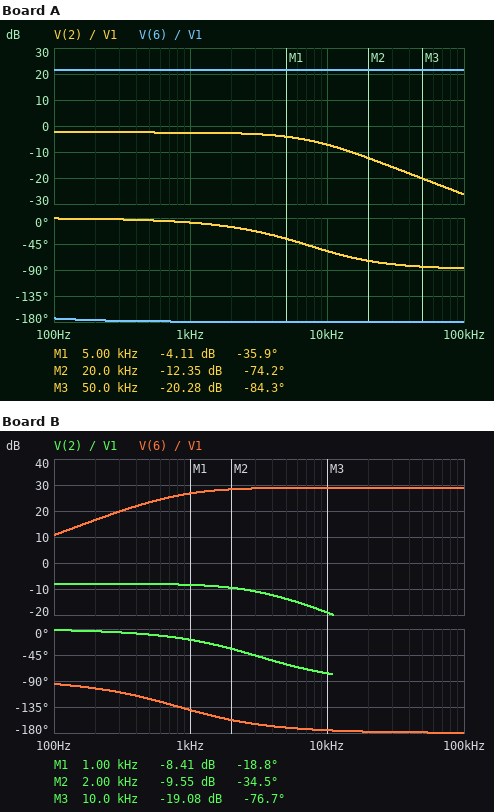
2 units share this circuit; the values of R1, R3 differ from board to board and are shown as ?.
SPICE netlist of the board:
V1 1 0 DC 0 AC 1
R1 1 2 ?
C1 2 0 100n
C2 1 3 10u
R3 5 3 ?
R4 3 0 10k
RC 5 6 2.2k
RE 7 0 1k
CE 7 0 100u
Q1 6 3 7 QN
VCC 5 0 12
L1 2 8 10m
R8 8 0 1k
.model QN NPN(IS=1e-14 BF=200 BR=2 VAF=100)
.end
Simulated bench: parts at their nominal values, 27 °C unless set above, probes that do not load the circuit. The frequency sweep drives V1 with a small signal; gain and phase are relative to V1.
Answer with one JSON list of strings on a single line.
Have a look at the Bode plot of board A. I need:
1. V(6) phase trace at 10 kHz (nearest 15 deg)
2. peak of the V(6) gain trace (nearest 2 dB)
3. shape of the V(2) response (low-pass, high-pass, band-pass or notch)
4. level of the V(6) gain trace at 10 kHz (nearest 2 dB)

["-180 deg", "22 dB", "low-pass", "22 dB"]
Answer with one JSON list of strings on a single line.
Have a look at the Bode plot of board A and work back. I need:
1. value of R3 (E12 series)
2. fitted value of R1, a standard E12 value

["150 kΩ", "330 Ω"]
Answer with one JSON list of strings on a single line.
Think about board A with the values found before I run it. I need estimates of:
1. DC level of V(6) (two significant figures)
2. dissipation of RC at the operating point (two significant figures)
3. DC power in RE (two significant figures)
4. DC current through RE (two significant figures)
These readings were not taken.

["12 V", "44 µW", "20 µW", "140 µA"]
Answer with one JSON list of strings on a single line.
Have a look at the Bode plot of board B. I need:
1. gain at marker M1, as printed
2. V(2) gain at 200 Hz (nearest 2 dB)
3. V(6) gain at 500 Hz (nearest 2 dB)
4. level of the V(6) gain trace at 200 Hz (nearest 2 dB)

["-8.41 dB", "-8 dB", "24 dB", "16 dB"]
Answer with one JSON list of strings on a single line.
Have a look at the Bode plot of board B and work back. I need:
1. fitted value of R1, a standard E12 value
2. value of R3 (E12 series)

["1.5 kΩ", "15 kΩ"]
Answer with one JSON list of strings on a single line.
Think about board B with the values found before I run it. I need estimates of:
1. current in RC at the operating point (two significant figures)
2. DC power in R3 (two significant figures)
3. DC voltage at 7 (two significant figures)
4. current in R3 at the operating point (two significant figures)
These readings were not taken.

["3.7 mA", "3.8 mW", "3.8 V", "500 µA"]
